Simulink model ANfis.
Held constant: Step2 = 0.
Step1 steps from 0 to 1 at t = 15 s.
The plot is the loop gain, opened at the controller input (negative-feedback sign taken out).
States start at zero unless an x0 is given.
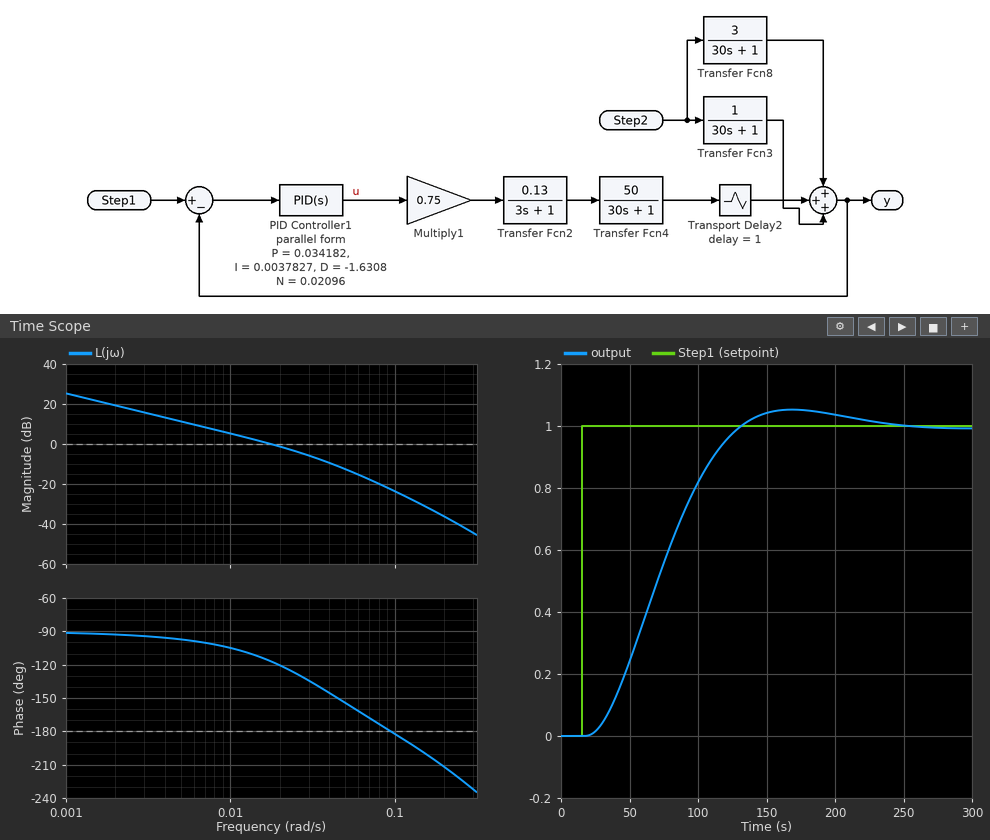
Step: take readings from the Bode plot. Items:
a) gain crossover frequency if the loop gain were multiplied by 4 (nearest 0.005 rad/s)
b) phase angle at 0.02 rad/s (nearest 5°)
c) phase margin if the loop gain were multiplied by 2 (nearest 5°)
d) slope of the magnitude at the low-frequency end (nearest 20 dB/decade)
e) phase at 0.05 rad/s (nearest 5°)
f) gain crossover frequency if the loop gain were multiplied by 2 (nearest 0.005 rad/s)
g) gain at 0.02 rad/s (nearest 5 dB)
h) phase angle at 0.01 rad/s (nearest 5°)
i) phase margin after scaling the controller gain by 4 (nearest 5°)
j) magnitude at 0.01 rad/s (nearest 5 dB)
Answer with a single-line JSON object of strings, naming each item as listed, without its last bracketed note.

{"gain crossover frequency if the loop gain were multiplied by 4": "0.050 rad/s", "phase angle at 0.02 rad/s": "-120°", "phase margin if the loop gain were multiplied by 2": "45°", "slope of the magnitude at the low-frequency end": "-20 dB/decade", "phase at 0.05 rad/s": "-155°", "gain crossover frequency if the loop gain were multiplied by 2": "0.030 rad/s", "gain at 0.02 rad/s": "0 dB", "phase angle at 0.01 rad/s": "-105°", "phase margin after scaling the controller gain by 4": "25°", "magnitude at 0.01 rad/s": "5 dB"}
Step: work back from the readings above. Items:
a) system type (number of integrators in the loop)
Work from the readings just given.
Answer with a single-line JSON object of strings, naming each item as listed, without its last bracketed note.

{"system type": "1"}
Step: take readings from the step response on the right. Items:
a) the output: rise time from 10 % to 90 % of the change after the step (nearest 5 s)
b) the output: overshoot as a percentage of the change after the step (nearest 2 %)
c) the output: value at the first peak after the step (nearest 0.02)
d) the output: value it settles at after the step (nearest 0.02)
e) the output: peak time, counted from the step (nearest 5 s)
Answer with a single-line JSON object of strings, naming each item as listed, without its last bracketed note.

{"the output: rise time from 10 % to 90 % of the change after the step": "75 s", "the output: overshoot as a percentage of the change after the step": "6 %", "the output: value at the first peak after the step": "1.06", "the output: value it settles at after the step": "1.00", "the output: peak time, counted from the step": "155 s"}
